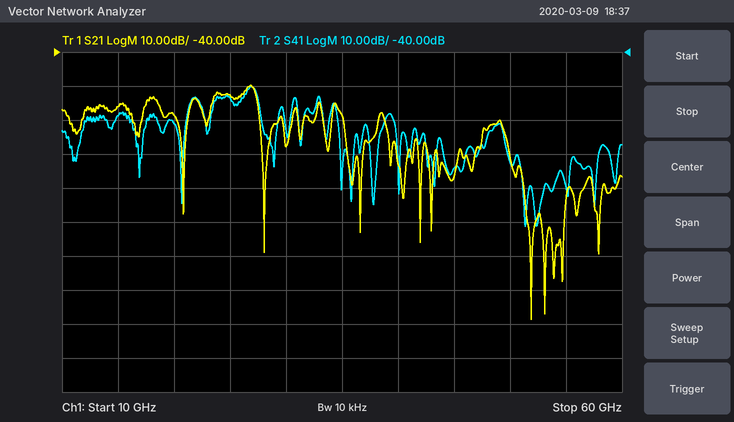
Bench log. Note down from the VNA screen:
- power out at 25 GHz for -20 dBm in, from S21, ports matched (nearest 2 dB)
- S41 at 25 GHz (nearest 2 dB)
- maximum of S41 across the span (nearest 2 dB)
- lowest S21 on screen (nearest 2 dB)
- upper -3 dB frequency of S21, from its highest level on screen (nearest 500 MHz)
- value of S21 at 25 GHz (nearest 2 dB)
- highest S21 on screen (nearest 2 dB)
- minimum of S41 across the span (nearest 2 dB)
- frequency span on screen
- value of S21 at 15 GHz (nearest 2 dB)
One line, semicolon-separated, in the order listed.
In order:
-72 dBm; -54 dB; -50 dB; -118 dB; 27.5 GHz; -52 dB; -50 dB; -92 dB; 50 GHz; -56 dB
